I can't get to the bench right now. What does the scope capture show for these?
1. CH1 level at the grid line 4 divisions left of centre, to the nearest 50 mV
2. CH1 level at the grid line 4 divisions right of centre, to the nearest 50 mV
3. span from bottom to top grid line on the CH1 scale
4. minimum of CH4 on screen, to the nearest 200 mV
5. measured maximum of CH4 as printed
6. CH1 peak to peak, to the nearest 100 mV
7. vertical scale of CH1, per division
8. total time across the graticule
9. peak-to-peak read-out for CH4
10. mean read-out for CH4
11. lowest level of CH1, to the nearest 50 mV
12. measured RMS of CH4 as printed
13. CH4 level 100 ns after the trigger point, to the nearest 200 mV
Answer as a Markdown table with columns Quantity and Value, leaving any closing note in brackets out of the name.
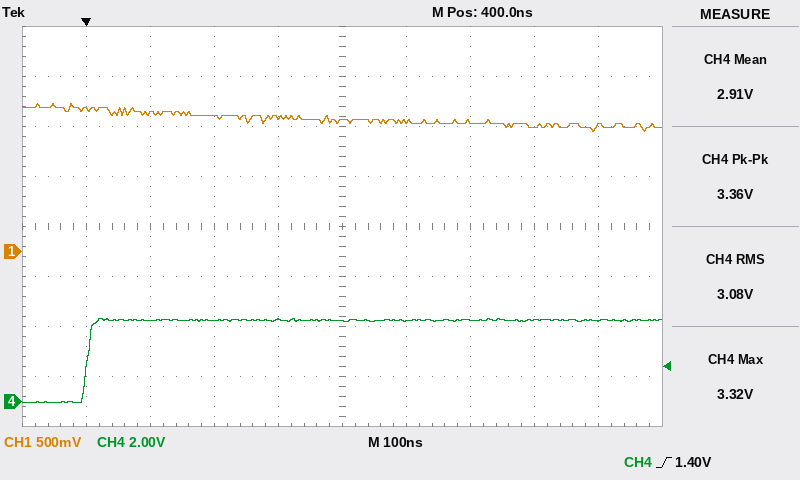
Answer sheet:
| Quantity | Value |
|---|---|
| CH1 level at the grid line 4 divisions left of centre, to the nearest 50 mV | 1.40 V |
| CH1 level at the grid line 4 divisions right of centre, to the nearest 50 mV | 1.25 V |
| span from bottom to top grid line on the CH1 scale | 4 V |
| minimum of CH4 on screen, to the nearest 200 mV | 0.0 V |
| measured maximum of CH4 as printed | 3.32 V |
| CH1 peak to peak, to the nearest 100 mV | 300 mV |
| vertical scale of CH1, per division | 500 mV |
| total time across the graticule | 1 µs |
| peak-to-peak read-out for CH4 | 3.36 V |
| mean read-out for CH4 | 2.91 V |
| lowest level of CH1, to the nearest 50 mV | 1.20 V |
| measured RMS of CH4 as printed | 3.08 V |
| CH4 level 100 ns after the trigger point, to the nearest 200 mV | 3.2 V |
